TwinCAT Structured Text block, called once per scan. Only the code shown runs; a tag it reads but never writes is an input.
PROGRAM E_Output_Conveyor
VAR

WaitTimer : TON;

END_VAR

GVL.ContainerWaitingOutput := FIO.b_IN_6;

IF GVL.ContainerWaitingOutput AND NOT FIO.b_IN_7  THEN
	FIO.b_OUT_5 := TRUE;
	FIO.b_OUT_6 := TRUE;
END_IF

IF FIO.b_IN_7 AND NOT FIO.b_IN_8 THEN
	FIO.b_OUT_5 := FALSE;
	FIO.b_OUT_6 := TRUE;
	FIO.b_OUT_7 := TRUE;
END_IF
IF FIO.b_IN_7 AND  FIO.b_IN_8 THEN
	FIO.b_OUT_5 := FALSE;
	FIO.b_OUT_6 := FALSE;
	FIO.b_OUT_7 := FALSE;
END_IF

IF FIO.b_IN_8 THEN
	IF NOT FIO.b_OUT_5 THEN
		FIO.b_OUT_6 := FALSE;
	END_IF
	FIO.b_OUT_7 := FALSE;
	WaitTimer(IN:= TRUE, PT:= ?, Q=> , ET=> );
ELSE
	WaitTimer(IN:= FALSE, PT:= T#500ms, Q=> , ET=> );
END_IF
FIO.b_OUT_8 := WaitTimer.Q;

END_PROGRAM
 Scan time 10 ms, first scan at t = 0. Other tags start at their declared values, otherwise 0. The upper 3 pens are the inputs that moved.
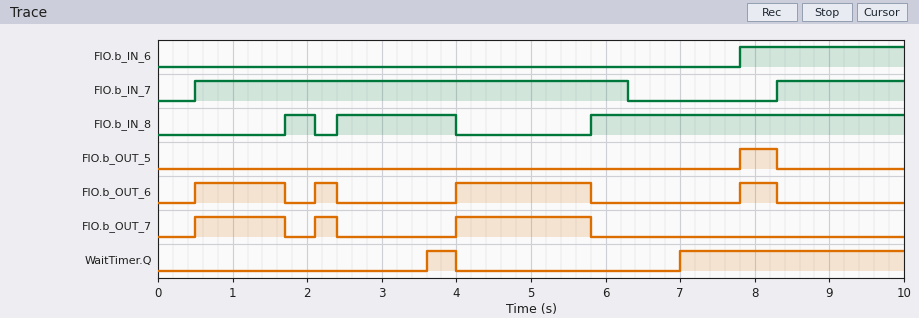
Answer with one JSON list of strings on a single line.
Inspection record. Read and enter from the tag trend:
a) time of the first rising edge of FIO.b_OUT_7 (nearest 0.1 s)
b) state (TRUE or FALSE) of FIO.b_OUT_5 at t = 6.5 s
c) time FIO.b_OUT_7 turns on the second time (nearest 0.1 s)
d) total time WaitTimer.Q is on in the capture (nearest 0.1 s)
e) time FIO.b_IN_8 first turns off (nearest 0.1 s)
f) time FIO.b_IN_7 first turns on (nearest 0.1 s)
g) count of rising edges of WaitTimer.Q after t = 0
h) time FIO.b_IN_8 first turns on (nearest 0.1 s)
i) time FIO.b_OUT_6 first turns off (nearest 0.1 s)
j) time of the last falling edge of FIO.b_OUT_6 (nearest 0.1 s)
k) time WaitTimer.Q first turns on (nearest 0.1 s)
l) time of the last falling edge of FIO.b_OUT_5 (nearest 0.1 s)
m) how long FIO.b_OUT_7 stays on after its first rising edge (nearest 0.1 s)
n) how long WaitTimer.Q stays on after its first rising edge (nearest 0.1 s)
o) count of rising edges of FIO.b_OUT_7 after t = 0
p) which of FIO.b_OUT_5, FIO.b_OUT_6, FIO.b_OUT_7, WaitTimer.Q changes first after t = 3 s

["0.5 s", "FALSE", "2.1 s", "3.4 s", "2.1 s", "0.5 s", "2", "1.7 s", "1.7 s", "8.3 s", "3.6 s", "8.3 s", "1.2 s", "0.4 s", "3", "WaitTimer.Q"]
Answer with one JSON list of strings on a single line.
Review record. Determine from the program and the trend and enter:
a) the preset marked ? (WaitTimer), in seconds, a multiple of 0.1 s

["1.2 s"]
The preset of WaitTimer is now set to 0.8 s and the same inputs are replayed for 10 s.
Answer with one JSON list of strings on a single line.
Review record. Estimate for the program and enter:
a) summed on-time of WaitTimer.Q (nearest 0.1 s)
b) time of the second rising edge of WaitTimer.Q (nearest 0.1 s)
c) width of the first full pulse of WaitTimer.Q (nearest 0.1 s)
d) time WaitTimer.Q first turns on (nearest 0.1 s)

["4.2 s", "6.6 s", "0.8 s", "3.2 s"]
